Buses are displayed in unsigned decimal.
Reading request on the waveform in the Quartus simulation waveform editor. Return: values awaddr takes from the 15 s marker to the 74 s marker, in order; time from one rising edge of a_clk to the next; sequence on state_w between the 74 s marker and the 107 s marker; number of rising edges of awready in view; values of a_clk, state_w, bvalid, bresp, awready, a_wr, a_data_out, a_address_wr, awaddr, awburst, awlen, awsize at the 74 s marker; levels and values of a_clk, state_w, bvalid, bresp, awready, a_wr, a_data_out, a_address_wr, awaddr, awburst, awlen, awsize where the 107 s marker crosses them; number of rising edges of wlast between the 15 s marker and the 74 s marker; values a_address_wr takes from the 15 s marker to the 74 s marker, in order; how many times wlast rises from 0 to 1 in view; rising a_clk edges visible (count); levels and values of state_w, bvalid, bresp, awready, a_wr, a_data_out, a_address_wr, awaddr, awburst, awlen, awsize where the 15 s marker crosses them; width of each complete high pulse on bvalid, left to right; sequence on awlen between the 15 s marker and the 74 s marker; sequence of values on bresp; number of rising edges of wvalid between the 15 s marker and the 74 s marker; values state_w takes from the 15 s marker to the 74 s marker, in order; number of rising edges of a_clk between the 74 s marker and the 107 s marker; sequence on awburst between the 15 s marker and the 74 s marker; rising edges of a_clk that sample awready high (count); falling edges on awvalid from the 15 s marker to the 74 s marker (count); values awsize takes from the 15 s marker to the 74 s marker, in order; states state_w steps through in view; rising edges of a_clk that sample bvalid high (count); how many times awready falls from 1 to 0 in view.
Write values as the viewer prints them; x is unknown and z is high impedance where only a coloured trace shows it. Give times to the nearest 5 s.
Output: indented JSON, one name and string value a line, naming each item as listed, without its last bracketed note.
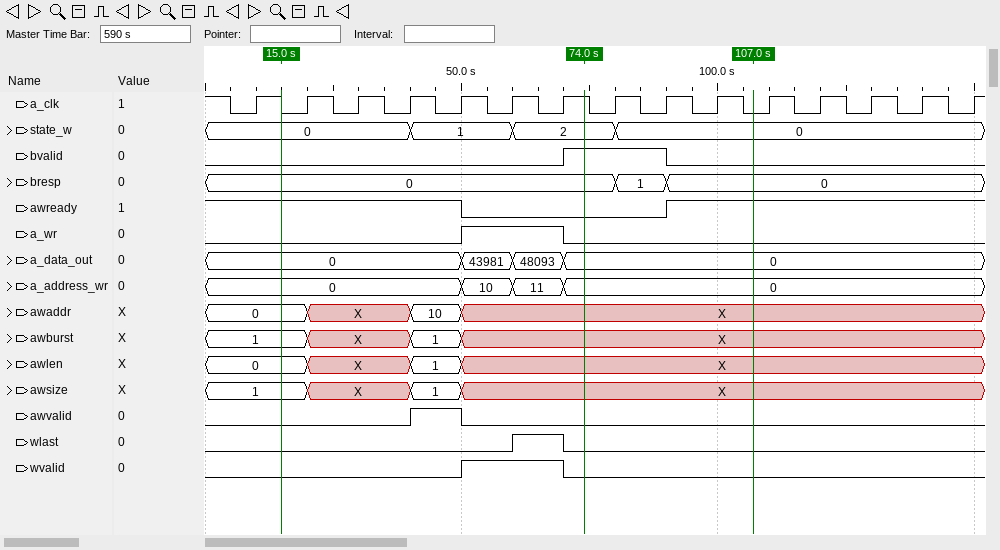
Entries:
{
  "values awaddr takes from the 15 s marker to the 74 s marker, in order": "0, X, 10, X",
  "time from one rising edge of a_clk to the next": "10 s",
  "sequence on state_w between the 74 s marker and the 107 s marker": "2, 0",
  "number of rising edges of awready in view": "1",
  "values of a_clk, state_w, bvalid, bresp, awready, a_wr, a_data_out, a_address_wr, awaddr, awburst, awlen, awsize at the 74 s marker": "a_clk=1, state_w=2, bvalid=1, bresp=0, awready=0, a_wr=0, a_data_out=0, a_address_wr=0, awaddr=X, awburst=X, awlen=X, awsize=X",
  "levels and values of a_clk, state_w, bvalid, bresp, awready, a_wr, a_data_out, a_address_wr, awaddr, awburst, awlen, awsize where the 107 s marker crosses them": "a_clk=0, state_w=0, bvalid=0, bresp=0, awready=1, a_wr=0, a_data_out=0, a_address_wr=0, awaddr=X, awburst=X, awlen=X, awsize=X",
  "number of rising edges of wlast between the 15 s marker and the 74 s marker": "1",
  "values a_address_wr takes from the 15 s marker to the 74 s marker, in order": "0, 10, 11, 0",
  "how many times wlast rises from 0 to 1 in view": "1",
  "rising a_clk edges visible": "15",
  "levels and values of state_w, bvalid, bresp, awready, a_wr, a_data_out, a_address_wr, awaddr, awburst, awlen, awsize where the 15 s marker crosses them": "state_w=0, bvalid=0, bresp=0, awready=1, a_wr=0, a_data_out=0, a_address_wr=0, awaddr=0, awburst=1, awlen=0, awsize=1",
  "width of each complete high pulse on bvalid, left to right": "20 s",
  "sequence on awlen between the 15 s marker and the 74 s marker": "0, X, 1, X",
  "sequence of values on bresp": "0, 1, 0",
  "number of rising edges of wvalid between the 15 s marker and the 74 s marker": "1",
  "values state_w takes from the 15 s marker to the 74 s marker, in order": "0, 1, 2",
  "number of rising edges of a_clk between the 74 s marker and the 107 s marker": "3",
  "sequence on awburst between the 15 s marker and the 74 s marker": "1, X, 1, X",
  "rising edges of a_clk that sample awready high": "11",
  "falling edges on awvalid from the 15 s marker to the 74 s marker": "1",
  "values awsize takes from the 15 s marker to the 74 s marker, in order": "1, X, 1, X",
  "states state_w steps through in view": "0, 1, 2, 0",
  "rising edges of a_clk that sample bvalid high": "2",
  "how many times awready falls from 1 to 0 in view": "1"
}
